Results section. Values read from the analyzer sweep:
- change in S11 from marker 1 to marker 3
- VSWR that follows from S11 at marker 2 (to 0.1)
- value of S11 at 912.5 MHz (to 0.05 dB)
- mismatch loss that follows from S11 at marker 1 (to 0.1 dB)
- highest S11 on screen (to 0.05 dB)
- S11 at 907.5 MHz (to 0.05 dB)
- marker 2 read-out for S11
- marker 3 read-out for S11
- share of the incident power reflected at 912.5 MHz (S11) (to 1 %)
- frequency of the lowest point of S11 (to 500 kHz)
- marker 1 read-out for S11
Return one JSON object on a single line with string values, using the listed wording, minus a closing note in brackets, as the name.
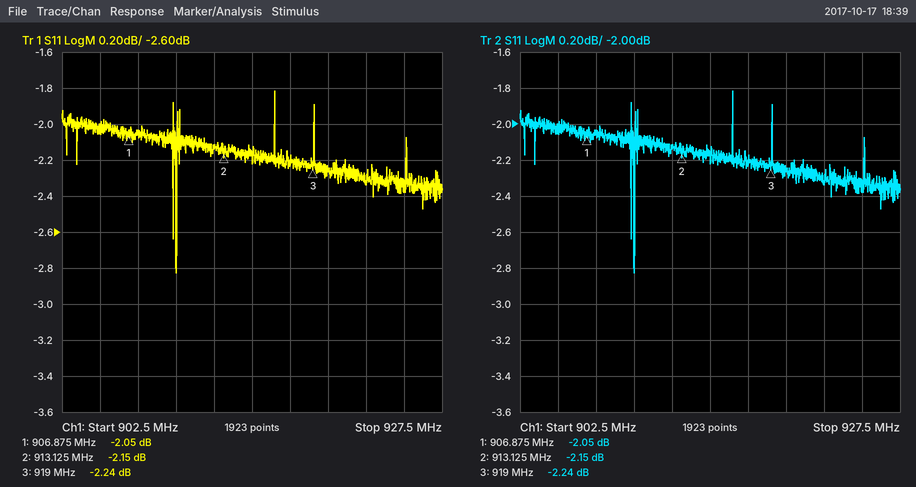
{"change in S11 from marker 1 to marker 3": "-0.19 dB", "VSWR that follows from S11 at marker 2": "8.1", "value of S11 at 912.5 MHz": "-2.15 dB", "mismatch loss that follows from S11 at marker 1": "4.2 dB", "highest S11 on screen": "-1.80 dB", "S11 at 907.5 MHz": "-2.05 dB", "marker 2 read-out for S11": "-2.15 dB", "marker 3 read-out for S11": "-2.24 dB", "share of the incident power reflected at 912.5 MHz (S11)": "61 %", "frequency of the lowest point of S11": "910.0 MHz", "marker 1 read-out for S11": "-2.05 dB"}
